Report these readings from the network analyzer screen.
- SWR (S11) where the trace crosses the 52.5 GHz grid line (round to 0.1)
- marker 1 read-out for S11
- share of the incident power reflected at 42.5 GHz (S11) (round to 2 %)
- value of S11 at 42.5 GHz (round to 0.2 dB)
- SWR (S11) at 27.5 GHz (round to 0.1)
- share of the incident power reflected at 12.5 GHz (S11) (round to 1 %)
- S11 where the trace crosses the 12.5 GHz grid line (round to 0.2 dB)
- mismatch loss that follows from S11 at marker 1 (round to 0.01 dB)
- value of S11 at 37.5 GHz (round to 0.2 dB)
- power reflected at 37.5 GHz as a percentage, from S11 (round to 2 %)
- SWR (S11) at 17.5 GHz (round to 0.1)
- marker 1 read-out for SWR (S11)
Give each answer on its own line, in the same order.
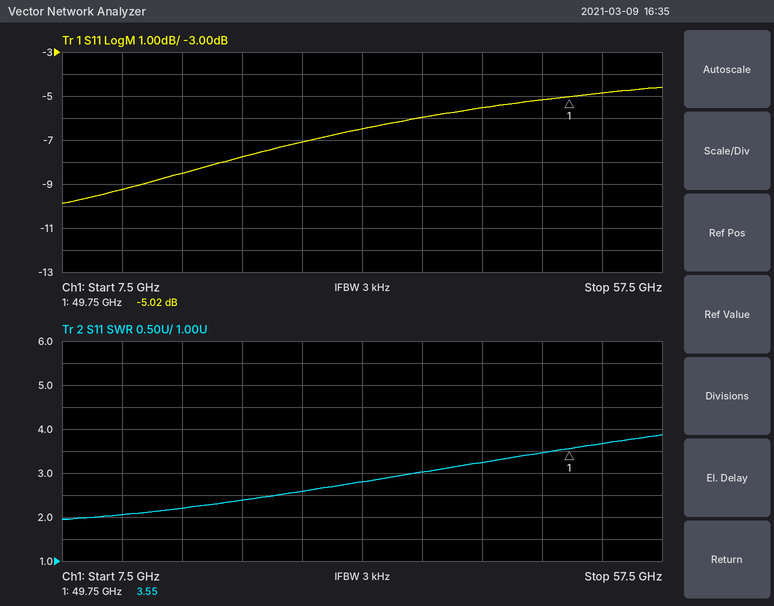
3.7
-5.02 dB
28 %
-5.6 dB
2.6
12 %
-9.2 dB
1.64 dB
-6.0 dB
26 %
2.2
3.55
